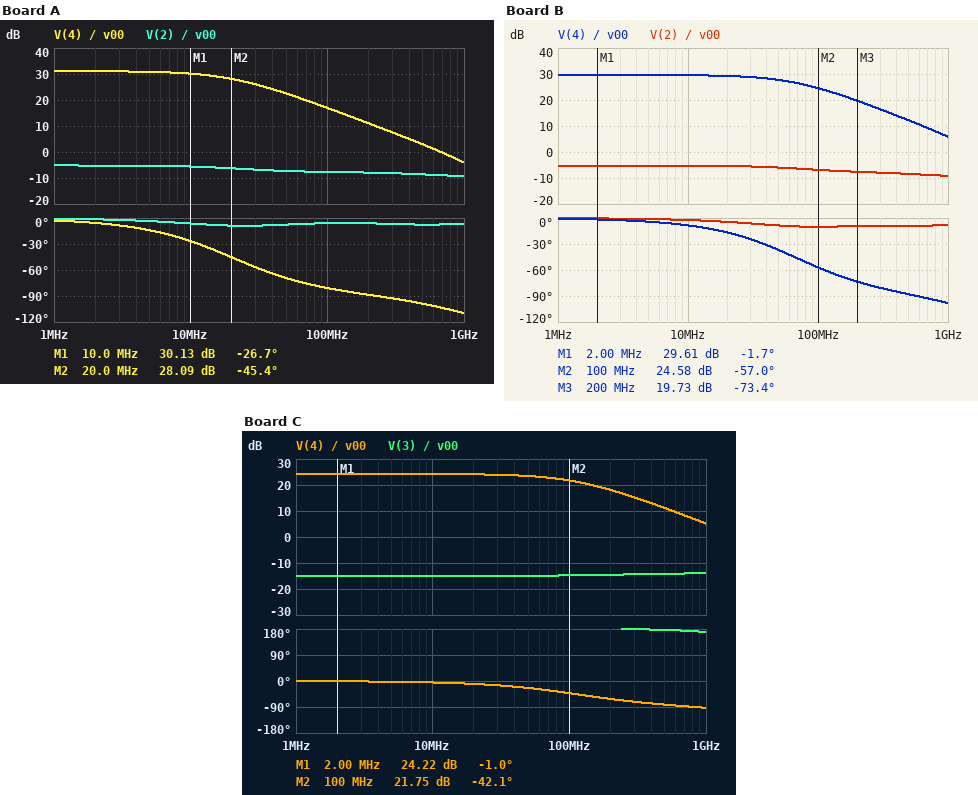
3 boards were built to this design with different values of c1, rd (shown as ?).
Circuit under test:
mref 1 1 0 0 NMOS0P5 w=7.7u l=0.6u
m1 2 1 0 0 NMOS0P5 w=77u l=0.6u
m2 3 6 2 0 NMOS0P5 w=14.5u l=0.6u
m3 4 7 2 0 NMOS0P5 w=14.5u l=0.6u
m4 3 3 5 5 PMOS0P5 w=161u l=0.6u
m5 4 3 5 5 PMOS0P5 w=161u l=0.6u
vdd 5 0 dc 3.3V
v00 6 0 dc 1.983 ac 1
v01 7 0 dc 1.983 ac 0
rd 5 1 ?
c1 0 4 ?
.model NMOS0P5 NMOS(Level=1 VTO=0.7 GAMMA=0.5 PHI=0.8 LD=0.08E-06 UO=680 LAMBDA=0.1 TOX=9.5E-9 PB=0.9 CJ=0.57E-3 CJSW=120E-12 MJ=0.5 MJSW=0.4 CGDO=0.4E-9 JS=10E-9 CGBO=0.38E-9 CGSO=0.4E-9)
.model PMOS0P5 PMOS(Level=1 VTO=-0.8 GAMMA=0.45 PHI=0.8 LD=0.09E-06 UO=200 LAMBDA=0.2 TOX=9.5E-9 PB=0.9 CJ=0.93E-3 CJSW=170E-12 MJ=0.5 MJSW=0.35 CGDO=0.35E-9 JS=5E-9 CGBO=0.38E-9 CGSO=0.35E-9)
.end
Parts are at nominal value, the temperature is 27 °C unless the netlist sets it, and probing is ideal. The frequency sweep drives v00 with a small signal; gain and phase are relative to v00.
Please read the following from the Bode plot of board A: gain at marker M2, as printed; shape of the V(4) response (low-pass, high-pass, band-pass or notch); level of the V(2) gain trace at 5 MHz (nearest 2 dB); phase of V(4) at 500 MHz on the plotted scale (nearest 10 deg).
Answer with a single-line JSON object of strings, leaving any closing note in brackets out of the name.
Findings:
{"gain at marker M2, as printed": "28.09 dB", "shape of the V(4) response": "low-pass", "level of the V(2) gain trace at 5 MHz": "-6 dB", "phase of V(4) at 500 MHz on the plotted scale": "-100 deg"}
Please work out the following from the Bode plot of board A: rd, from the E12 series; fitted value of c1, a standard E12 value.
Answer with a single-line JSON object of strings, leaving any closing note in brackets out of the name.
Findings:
{"rd, from the E12 series": "56 kΩ", "fitted value of c1, a standard E12 value": "330 fF"}
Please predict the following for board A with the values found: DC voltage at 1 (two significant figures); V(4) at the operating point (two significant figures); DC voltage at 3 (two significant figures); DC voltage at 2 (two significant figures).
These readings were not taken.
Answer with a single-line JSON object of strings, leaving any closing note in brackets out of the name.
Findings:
{"DC voltage at 1": "840 mV", "V(4) at the operating point": "2.4 V", "DC voltage at 3": "2.4 V", "DC voltage at 2": "870 mV"}
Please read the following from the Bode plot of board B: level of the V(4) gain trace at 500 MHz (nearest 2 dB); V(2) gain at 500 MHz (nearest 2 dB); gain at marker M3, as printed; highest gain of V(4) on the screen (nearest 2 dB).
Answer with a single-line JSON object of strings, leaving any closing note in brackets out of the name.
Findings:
{"level of the V(4) gain trace at 500 MHz": "12 dB", "V(2) gain at 500 MHz": "-8 dB", "gain at marker M3, as printed": "19.73 dB", "highest gain of V(4) on the screen": "30 dB"}
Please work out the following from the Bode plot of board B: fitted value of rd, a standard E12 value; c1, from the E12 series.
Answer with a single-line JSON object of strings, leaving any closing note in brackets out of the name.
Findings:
{"fitted value of rd, a standard E12 value": "39 kΩ", "c1, from the E12 series": "68 fF"}
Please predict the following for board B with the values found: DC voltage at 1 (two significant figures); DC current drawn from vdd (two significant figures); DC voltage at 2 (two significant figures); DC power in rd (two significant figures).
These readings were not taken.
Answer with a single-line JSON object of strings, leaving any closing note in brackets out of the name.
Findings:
{"DC voltage at 1": "860 mV", "DC current drawn from vdd": "690 µA", "DC voltage at 2": "830 mV", "DC power in rd": "150 µW"}
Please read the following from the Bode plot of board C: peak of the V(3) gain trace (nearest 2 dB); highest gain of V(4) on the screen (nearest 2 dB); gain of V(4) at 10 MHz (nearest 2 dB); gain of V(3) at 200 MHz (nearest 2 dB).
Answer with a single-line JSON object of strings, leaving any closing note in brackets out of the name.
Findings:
{"peak of the V(3) gain trace": "-14 dB", "highest gain of V(4) on the screen": "24 dB", "gain of V(4) at 10 MHz": "24 dB", "gain of V(3) at 200 MHz": "-14 dB"}
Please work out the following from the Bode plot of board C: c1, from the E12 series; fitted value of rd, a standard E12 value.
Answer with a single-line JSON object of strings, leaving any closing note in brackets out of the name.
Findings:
{"c1, from the E12 series": "270 fF", "fitted value of rd, a standard E12 value": "10 kΩ"}
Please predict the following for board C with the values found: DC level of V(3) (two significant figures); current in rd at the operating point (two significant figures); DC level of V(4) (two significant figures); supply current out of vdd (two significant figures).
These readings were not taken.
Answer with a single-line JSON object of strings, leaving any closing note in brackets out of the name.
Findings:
{"DC level of V(3)": "2.2 V", "current in rd at the operating point": "230 µA", "DC level of V(4)": "2.2 V", "supply current out of vdd": "2.4 mA"}
